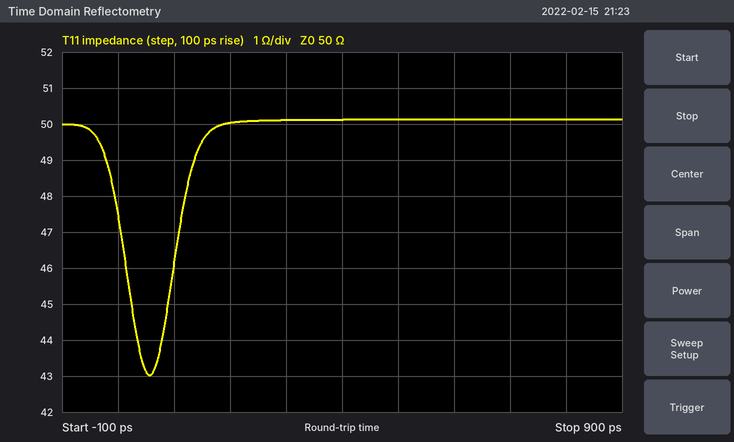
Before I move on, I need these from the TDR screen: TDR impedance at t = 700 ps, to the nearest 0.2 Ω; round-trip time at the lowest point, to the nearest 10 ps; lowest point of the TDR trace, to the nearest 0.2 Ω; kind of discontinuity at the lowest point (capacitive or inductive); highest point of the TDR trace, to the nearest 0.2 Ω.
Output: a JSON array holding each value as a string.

["50.2 Ω", "60 ps", "43.0 Ω", "capacitive", "50.2 Ω"]
